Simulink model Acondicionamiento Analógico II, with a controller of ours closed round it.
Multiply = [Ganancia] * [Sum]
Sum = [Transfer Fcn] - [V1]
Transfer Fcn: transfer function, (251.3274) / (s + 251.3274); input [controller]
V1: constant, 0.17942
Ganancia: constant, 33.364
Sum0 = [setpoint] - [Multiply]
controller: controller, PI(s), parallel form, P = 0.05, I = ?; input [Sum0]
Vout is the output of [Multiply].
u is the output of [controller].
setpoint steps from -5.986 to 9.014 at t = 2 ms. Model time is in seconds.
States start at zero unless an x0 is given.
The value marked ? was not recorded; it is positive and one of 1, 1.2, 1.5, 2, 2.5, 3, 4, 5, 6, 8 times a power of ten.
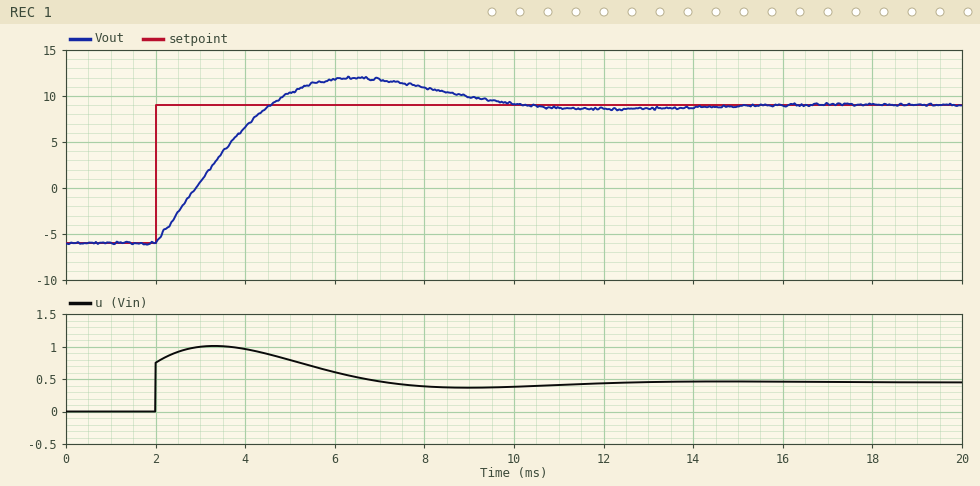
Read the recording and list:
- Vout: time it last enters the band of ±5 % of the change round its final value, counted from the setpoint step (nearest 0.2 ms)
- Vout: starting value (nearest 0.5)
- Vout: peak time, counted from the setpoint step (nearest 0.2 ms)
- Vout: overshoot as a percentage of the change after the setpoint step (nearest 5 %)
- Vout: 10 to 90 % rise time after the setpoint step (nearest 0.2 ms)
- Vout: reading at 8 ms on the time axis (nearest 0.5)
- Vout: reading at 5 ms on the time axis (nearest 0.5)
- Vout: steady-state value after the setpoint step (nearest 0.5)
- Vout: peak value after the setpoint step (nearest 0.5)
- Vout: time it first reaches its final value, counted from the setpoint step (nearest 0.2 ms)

7.2 ms
-6.0
4.4 ms
20 %
2.0 ms
11.0
10.5
9.0
12.0
2.6 ms
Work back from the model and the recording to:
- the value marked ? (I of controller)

50
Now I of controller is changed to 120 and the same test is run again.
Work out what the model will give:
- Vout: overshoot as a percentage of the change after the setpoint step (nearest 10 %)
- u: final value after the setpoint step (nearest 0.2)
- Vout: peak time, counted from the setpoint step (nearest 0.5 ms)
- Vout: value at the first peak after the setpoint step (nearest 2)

40 %
0.4
3.0 ms
14
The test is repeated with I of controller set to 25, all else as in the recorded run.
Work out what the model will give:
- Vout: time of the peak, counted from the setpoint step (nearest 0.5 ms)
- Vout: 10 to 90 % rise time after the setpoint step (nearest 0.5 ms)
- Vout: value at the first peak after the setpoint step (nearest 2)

6.5 ms
3.0 ms
10
